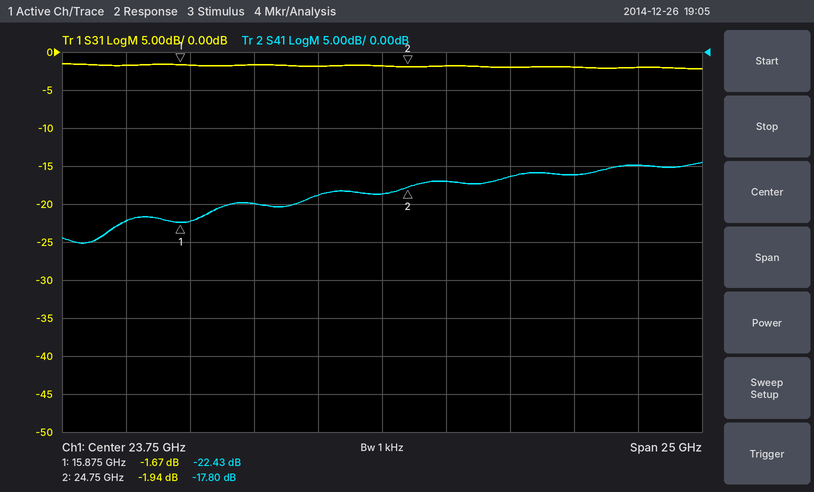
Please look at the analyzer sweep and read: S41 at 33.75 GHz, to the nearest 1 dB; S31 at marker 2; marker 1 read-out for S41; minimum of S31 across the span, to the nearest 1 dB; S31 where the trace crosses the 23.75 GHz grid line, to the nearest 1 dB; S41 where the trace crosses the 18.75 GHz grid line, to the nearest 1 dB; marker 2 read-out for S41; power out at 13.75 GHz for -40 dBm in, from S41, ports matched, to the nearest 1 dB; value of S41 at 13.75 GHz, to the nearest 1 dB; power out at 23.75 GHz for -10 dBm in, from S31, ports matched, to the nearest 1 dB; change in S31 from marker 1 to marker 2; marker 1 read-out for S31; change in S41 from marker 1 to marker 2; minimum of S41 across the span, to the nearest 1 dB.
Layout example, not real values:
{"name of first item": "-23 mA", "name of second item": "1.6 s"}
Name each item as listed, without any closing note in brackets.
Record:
{"S41 at 33.75 GHz, to the nearest 1 dB": "-15 dB", "S31 at marker 2": "-1.94 dB", "marker 1 read-out for S41": "-22.43 dB", "minimum of S31 across the span, to the nearest 1 dB": "-2 dB", "S31 where the trace crosses the 23.75 GHz grid line, to the nearest 1 dB": "-2 dB", "S41 where the trace crosses the 18.75 GHz grid line, to the nearest 1 dB": "-20 dB", "marker 2 read-out for S41": "-17.80 dB", "power out at 13.75 GHz for -40 dBm in, from S41, ports matched, to the nearest 1 dB": "-62 dBm", "value of S41 at 13.75 GHz, to the nearest 1 dB": "-22 dB", "power out at 23.75 GHz for -10 dBm in, from S31, ports matched, to the nearest 1 dB": "-12 dBm", "change in S31 from marker 1 to marker 2": "-0.27 dB", "marker 1 read-out for S31": "-1.67 dB", "change in S41 from marker 1 to marker 2": "4.63 dB", "minimum of S41 across the span, to the nearest 1 dB": "-25 dB"}
